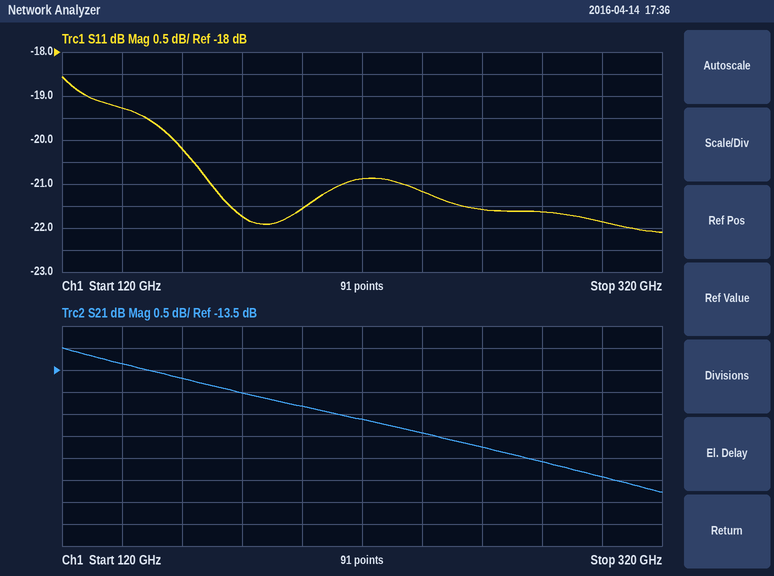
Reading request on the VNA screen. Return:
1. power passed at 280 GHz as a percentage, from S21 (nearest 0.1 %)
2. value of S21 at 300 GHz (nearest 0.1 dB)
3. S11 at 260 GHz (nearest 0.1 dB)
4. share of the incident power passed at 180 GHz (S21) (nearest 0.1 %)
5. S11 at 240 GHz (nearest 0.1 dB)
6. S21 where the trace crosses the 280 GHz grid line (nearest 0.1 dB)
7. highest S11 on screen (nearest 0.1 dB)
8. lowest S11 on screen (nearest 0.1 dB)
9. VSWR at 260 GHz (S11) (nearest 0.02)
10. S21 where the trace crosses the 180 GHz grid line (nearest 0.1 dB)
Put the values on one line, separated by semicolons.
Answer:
2.8 %; -15.9 dB; -21.6 dB; 4.0 %; -21.2 dB; -15.6 dB; -18.6 dB; -22.1 dB; 1.18; -14.0 dB
